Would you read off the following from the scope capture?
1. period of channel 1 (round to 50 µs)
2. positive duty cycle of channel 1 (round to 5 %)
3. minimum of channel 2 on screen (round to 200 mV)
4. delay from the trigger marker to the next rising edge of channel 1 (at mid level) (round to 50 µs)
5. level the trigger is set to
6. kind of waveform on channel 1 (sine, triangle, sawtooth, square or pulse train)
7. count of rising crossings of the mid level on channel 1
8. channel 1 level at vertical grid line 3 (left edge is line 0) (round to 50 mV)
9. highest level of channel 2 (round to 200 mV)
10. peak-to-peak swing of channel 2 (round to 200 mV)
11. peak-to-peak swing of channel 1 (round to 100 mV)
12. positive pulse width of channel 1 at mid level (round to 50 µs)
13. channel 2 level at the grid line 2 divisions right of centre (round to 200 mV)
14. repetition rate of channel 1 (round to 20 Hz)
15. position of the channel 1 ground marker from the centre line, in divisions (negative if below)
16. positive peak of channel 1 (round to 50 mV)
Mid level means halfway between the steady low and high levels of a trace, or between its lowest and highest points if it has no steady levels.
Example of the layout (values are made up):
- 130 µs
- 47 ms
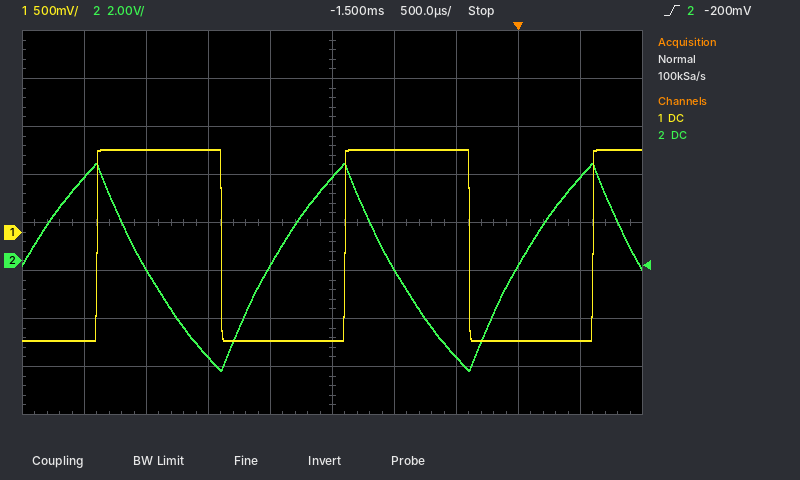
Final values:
- 2.00 ms
- 50 %
- -4.6 V
- 600 µs
- -200 mV
- square
- 3
- 850 mV
- 4.0 V
- 8.6 V
- 2.00 V
- 1.00 ms
- -4.0 V
- 500 Hz
- -0.2 div
- 850 mV
